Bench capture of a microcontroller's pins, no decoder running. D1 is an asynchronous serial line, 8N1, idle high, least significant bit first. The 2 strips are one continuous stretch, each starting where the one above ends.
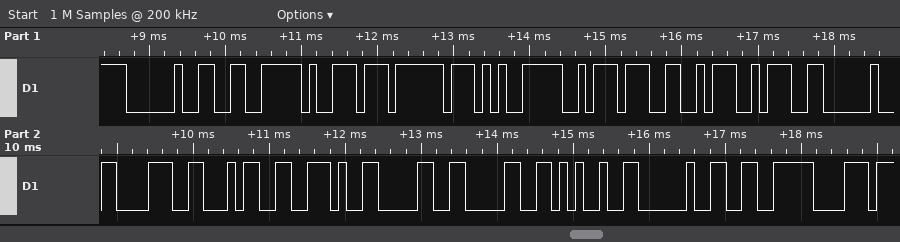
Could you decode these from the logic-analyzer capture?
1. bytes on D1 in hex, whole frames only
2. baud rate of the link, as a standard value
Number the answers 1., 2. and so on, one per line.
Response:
1. 20 E6 B9 BF E5 BA A6 3A 20 38 34 2E 30 30 25 20 E6 B8
2. 9600 baud
